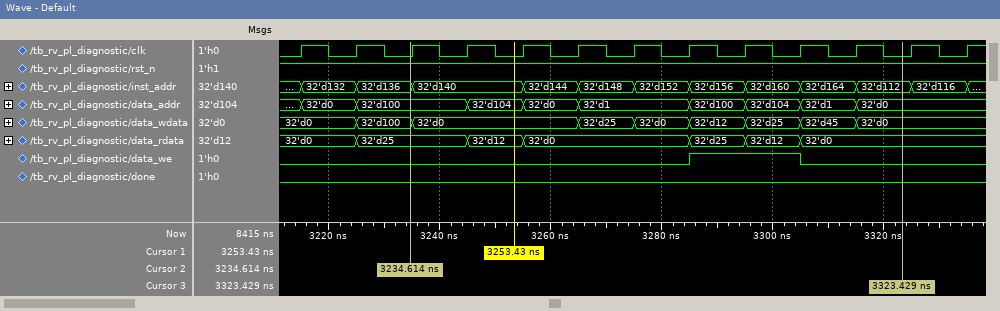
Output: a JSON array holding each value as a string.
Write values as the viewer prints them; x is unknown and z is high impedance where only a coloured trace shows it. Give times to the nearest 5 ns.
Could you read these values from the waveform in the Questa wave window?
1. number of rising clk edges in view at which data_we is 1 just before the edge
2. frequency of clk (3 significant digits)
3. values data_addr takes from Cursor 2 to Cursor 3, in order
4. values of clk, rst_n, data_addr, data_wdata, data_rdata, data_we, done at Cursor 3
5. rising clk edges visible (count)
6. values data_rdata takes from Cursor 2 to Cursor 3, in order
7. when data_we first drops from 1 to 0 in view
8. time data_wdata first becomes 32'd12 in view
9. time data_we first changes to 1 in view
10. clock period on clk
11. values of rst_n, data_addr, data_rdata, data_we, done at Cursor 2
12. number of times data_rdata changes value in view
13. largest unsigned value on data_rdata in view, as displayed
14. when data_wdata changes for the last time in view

["2", "100 MHz", "32'd100, 32'd104, 32'd0, 32'd1, 32'd100, 32'd104, 32'd1, 32'd0", "clk=0, rst_n=1, data_addr=32'd0, data_wdata=32'd0, data_rdata=32'd0, data_we=0, done=0", "13", "32'd25, 32'd12, 32'd0, 32'd25, 32'd12, 32'd0", "3305 ns", "3285 ns", "3285 ns", "10 ns", "rst_n=1, data_addr=32'd100, data_rdata=32'd25, data_we=0, done=0", "6", "32'd25", "3315 ns"]
